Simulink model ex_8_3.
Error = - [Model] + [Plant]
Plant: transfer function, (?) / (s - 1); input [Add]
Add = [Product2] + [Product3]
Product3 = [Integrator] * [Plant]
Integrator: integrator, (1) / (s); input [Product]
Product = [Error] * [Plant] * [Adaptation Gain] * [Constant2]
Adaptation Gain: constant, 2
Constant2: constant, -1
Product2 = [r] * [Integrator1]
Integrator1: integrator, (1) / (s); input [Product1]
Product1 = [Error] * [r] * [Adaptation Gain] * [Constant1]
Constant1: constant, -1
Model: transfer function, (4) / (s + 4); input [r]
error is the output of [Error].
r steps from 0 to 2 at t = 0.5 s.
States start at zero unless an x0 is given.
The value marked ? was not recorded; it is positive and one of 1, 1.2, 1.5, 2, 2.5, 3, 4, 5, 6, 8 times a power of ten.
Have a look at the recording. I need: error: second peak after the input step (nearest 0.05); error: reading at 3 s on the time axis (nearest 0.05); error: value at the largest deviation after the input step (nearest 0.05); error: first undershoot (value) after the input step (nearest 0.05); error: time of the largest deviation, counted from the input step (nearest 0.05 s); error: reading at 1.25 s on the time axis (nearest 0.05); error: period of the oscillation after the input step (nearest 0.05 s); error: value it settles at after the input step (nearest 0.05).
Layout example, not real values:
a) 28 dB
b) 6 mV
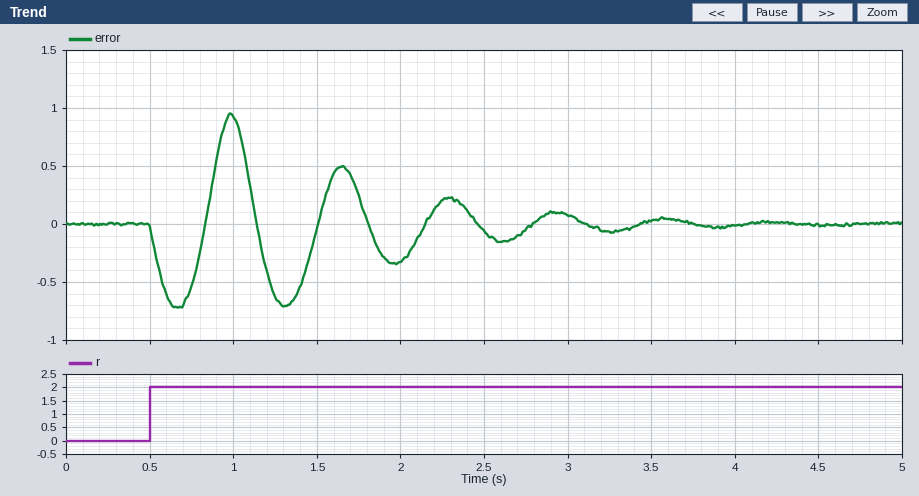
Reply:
a) 0.50
b) 0.10
c) 0.95
d) -0.70
e) 0.50 s
f) -0.60
g) 0.65 s
h) 0.00
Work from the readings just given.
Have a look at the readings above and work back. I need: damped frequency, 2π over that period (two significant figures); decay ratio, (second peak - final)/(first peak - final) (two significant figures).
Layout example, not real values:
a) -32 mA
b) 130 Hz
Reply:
a) 9.7 rad/s
b) 0.53
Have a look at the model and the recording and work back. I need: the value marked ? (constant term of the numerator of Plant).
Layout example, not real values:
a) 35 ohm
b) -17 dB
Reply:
a) 6
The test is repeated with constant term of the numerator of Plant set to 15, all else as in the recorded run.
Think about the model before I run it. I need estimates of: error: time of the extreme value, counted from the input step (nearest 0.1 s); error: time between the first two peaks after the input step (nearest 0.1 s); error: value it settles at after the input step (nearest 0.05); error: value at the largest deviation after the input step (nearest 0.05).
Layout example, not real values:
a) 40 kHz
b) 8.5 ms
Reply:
a) 0.3 s
b) 0.4 s
c) 0.00
d) 0.70
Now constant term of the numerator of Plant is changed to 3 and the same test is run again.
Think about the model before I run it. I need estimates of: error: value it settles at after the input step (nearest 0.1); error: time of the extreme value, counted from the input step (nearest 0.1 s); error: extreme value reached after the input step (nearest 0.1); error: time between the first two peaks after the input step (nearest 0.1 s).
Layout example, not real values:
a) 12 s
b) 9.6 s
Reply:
a) 0.0
b) 0.6 s
c) 1.2
d) 0.9 s
